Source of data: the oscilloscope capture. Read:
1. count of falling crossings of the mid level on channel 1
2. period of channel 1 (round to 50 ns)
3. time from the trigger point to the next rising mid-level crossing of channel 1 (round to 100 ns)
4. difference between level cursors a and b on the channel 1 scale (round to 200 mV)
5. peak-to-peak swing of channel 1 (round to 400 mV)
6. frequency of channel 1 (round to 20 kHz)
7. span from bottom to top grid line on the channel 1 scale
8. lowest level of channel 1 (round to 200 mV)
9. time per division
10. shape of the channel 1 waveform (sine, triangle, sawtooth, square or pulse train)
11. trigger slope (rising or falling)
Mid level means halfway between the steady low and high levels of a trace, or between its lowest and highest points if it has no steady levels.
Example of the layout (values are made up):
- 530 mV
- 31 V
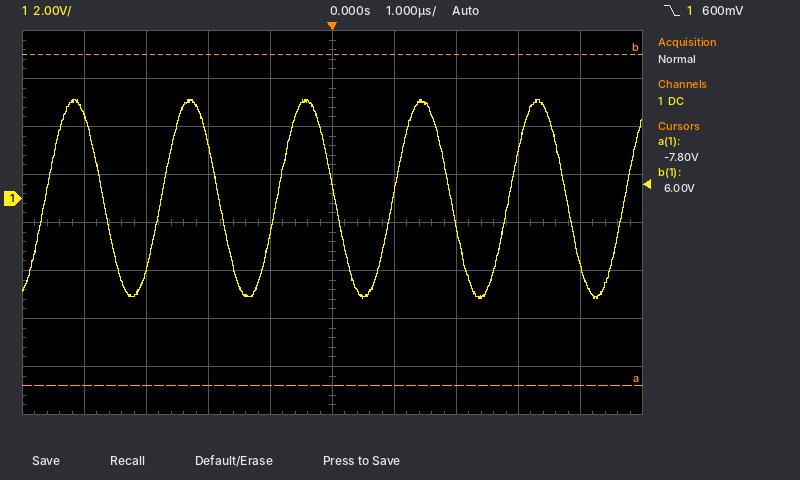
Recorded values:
- 5
- 1.85 µs
- 1.0 µs
- 13.8 V
- 8.4 V
- 540 kHz
- 16 V
- -4.2 V
- 1 µs
- sine
- falling
